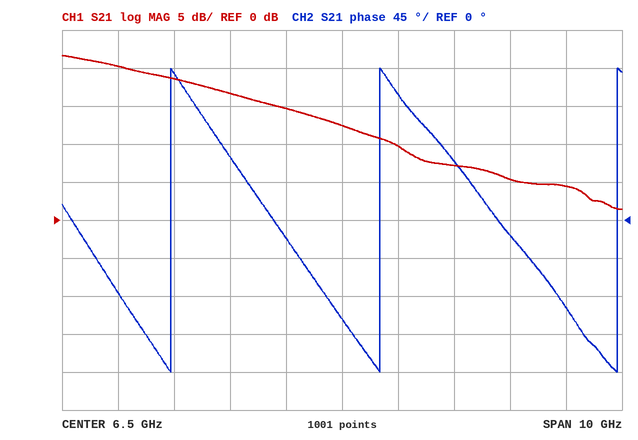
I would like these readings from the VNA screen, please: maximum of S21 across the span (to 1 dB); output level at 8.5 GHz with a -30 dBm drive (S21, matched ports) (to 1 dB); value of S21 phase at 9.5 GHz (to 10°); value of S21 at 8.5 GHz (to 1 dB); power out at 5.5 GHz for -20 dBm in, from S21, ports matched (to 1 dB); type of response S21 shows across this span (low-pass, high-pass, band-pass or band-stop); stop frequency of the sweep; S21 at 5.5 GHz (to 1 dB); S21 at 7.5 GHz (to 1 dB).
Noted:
22 dB
-23 dBm
-20°
7 dB
-5 dBm
low-pass
11.5 GHz
15 dB
10 dB
